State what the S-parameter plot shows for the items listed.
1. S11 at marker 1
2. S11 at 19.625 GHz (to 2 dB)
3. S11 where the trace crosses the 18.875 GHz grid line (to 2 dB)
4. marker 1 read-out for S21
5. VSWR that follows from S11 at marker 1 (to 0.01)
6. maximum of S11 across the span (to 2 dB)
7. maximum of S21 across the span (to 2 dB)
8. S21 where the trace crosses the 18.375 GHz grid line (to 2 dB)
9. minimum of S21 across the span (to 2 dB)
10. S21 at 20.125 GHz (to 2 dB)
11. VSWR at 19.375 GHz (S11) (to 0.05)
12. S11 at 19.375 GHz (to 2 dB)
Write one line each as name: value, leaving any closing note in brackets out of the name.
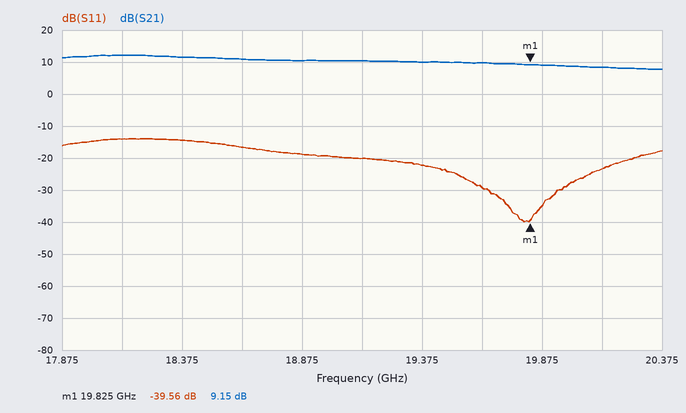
S11 at marker 1: -39.56 dB
S11 at 19.625 GHz: -30 dB
S11 where the trace crosses the 18.875 GHz grid line: -18 dB
marker 1 read-out for S21: 9.15 dB
VSWR that follows from S11 at marker 1: 1.02
maximum of S11 across the span: -14 dB
maximum of S21 across the span: 12 dB
S21 where the trace crosses the 18.375 GHz grid line: 12 dB
minimum of S21 across the span: 8 dB
S21 at 20.125 GHz: 8 dB
VSWR at 19.375 GHz (S11): 1.15
S11 at 19.375 GHz: -22 dB
